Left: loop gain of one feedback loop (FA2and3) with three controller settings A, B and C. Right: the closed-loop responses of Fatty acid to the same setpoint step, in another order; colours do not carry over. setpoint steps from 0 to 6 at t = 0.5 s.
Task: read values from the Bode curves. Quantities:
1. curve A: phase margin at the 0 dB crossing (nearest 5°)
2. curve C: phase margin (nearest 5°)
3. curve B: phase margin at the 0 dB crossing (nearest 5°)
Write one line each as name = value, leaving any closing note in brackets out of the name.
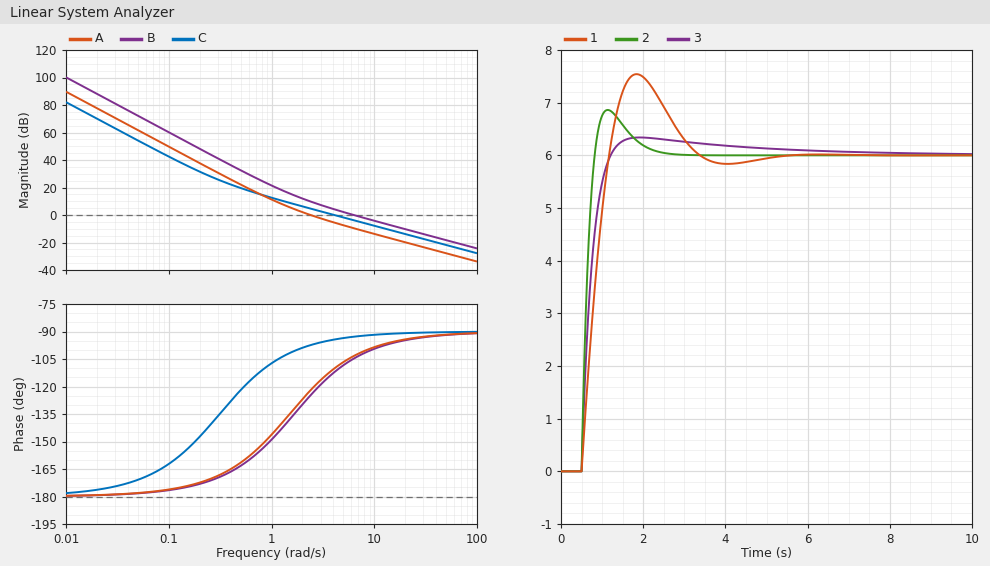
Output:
curve A: phase margin at the 0 dB crossing = 60°
curve C: phase margin = 85°
curve B: phase margin at the 0 dB crossing = 75°
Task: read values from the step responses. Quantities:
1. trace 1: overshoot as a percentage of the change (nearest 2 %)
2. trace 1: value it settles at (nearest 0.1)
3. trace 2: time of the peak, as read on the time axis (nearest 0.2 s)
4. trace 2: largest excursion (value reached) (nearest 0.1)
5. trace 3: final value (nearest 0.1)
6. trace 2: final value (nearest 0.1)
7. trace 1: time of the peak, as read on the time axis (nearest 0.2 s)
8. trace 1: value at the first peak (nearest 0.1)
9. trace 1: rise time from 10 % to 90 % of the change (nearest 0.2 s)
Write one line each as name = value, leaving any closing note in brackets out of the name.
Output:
trace 1: overshoot as a percentage of the change = 26 %
trace 1: value it settles at = 6.0
trace 2: time of the peak, as read on the time axis = 1.2 s
trace 2: largest excursion (value reached) = 6.9
trace 3: final value = 6.0
trace 2: final value = 6.0
trace 1: time of the peak, as read on the time axis = 1.8 s
trace 1: value at the first peak = 7.5
trace 1: rise time from 10 % to 90 % of the change = 0.6 s
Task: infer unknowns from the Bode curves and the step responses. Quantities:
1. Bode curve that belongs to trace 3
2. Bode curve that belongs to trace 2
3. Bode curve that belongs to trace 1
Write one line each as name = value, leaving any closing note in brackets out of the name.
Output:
Bode curve that belongs to trace 3 = C
Bode curve that belongs to trace 2 = B
Bode curve that belongs to trace 1 = A
